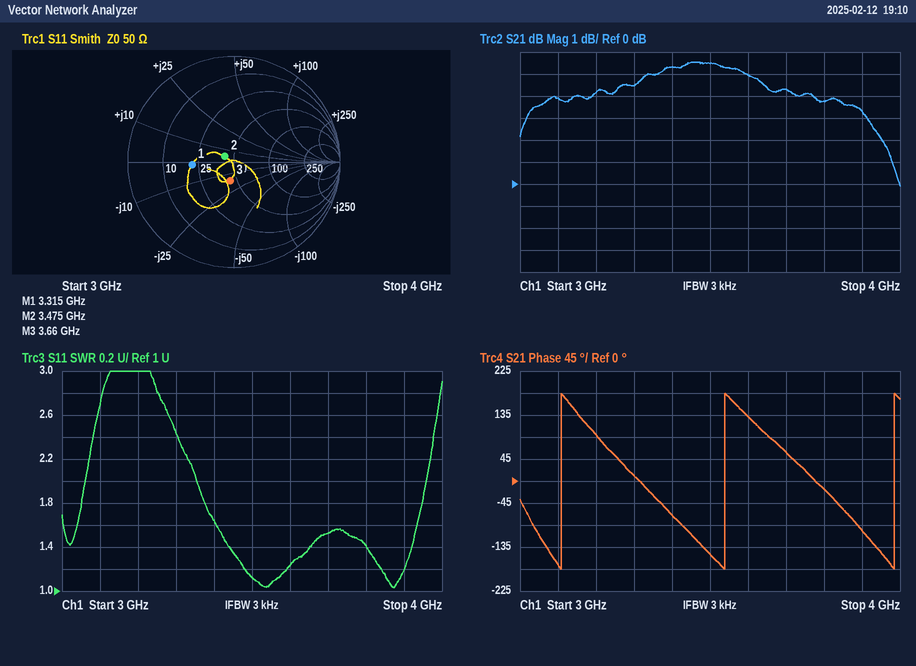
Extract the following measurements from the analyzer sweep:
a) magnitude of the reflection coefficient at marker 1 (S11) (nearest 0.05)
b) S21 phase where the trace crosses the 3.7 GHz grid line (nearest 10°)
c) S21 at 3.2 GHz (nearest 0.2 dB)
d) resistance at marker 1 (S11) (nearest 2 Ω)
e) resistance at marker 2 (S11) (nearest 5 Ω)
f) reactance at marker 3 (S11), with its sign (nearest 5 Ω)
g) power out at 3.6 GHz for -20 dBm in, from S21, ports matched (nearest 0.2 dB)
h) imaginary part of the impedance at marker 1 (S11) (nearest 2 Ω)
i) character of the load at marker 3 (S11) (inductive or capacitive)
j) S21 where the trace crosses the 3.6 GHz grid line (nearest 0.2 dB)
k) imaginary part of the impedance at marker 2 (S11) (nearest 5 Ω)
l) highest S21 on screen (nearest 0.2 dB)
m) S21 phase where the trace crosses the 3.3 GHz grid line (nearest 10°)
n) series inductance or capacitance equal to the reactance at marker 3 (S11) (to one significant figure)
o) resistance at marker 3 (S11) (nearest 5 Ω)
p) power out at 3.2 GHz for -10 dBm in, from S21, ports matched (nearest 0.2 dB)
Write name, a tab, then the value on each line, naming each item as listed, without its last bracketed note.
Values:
magnitude of the reflection coefficient at marker 1 (S11)	0.40
S21 phase where the trace crosses the 3.7 GHz grid line	60°
S21 at 3.2 GHz	4.2 dB
resistance at marker 1 (S11)	22 Ω
resistance at marker 2 (S11)	40 Ω
reactance at marker 3 (S11), with its sign	-15 Ω
power out at 3.6 GHz for -20 dBm in, from S21, ports matched	-15.0 dBm
imaginary part of the impedance at marker 1 (S11)	-2 Ω
character of the load at marker 3 (S11)	capacitive
S21 where the trace crosses the 3.6 GHz grid line	5.0 dB
imaginary part of the impedance at marker 2 (S11)	+5 Ω
highest S21 on screen	5.6 dB
S21 phase where the trace crosses the 3.3 GHz grid line	10°
series inductance or capacitance equal to the reactance at marker 3 (S11)	3 pF
resistance at marker 3 (S11)	45 Ω
power out at 3.2 GHz for -10 dBm in, from S21, ports matched	-5.8 dBm
